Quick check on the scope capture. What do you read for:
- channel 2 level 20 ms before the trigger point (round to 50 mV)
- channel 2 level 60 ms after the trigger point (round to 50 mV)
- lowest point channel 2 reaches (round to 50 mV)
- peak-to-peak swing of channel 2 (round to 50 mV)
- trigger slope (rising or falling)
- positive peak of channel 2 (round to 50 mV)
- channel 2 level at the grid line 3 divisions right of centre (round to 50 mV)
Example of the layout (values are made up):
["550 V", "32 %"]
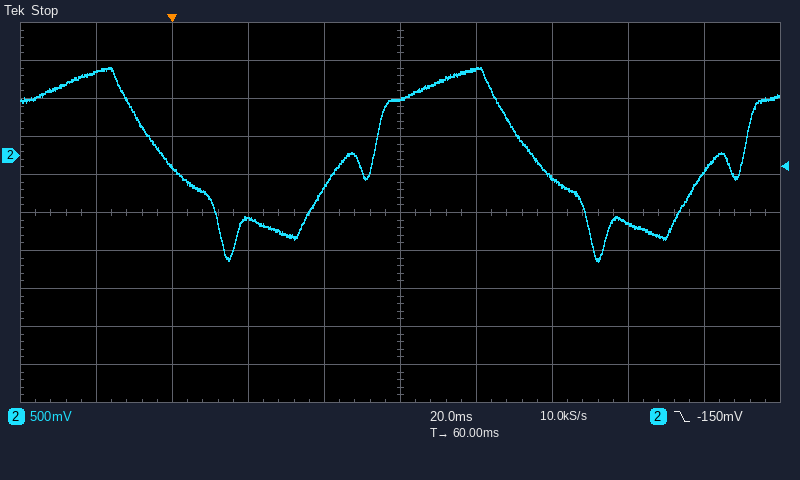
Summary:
["1.10 V", "750 mV", "-1.40 V", "2.55 V", "falling", "1.15 V", "-900 mV"]
